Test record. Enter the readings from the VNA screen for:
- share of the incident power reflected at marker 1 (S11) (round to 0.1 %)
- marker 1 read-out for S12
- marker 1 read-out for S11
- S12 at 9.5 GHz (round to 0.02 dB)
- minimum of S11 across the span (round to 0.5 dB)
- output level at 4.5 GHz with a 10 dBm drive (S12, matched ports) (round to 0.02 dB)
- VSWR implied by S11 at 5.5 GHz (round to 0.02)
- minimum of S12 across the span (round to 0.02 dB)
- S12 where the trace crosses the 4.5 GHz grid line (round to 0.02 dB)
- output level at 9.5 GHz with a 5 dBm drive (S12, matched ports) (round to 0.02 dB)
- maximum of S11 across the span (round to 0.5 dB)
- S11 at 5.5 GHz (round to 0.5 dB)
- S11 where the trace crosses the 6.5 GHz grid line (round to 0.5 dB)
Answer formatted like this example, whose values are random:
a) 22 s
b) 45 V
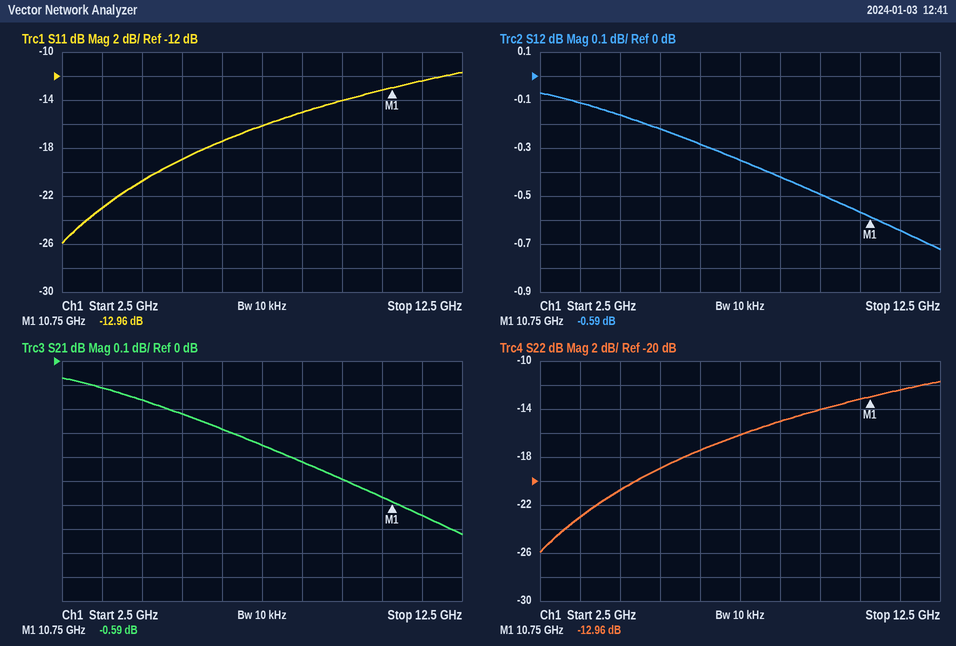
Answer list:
a) 5.1 %
b) -0.59 dB
c) -12.96 dB
d) -0.50 dB
e) -26.0 dB
f) 9.84 dBm
g) 1.26
h) -0.72 dB
i) -0.16 dB
j) 4.50 dBm
k) -11.5 dB
l) -19.0 dB
m) -17.5 dB
